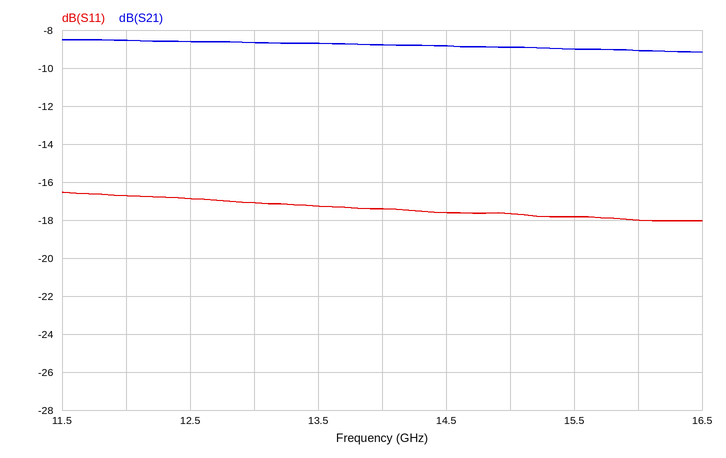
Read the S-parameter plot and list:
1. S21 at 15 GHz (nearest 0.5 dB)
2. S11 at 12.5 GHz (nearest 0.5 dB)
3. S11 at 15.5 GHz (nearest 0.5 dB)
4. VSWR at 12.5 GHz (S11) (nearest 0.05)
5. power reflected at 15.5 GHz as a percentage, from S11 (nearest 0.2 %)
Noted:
-9.0 dB
-17.0 dB
-18.0 dB
1.35
1.6 %
